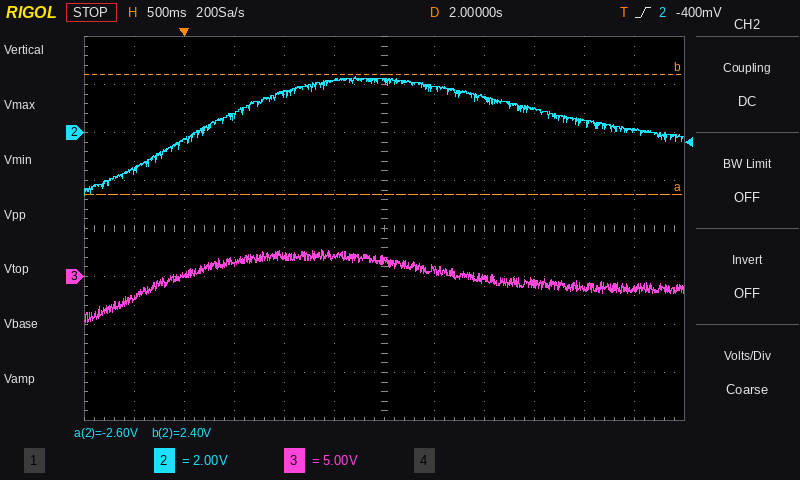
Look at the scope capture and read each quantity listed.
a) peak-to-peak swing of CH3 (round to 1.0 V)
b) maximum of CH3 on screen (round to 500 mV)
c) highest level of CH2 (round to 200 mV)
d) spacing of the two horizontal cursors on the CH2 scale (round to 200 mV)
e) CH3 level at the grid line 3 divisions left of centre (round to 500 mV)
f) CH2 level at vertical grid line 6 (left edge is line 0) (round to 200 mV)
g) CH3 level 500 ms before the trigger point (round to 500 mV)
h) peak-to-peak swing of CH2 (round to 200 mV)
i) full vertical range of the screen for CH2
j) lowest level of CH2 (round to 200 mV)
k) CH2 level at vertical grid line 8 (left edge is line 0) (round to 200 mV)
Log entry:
8.0 V
3.0 V
2.4 V
5.0 V
1.5 V
2.2 V
-2.0 V
5.0 V
16 V
-2.6 V
1.4 V
